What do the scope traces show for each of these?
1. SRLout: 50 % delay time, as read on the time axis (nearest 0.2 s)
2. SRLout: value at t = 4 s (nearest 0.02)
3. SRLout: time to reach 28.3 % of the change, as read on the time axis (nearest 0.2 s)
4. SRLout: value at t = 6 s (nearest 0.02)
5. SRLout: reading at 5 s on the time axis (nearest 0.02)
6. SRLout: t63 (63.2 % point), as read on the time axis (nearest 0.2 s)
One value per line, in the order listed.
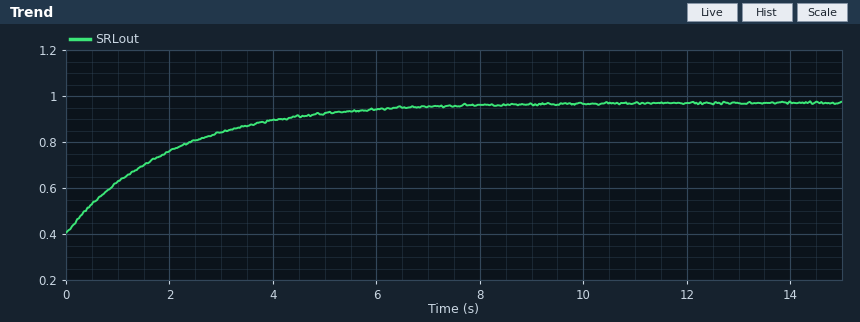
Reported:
1.4 s
0.90
0.6 s
0.94
0.92
2.0 s
